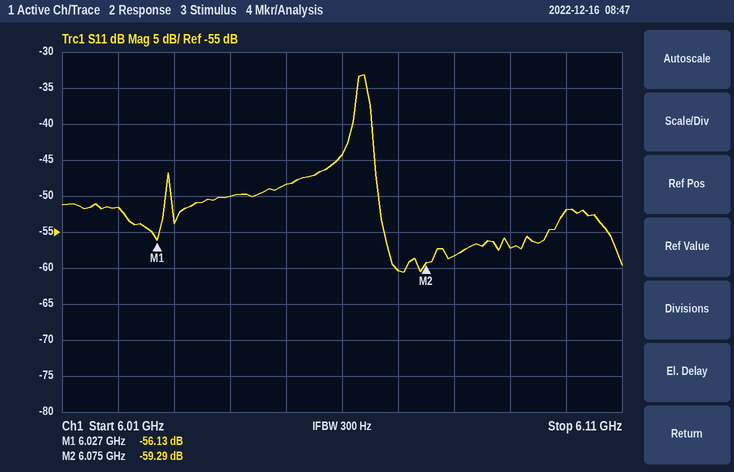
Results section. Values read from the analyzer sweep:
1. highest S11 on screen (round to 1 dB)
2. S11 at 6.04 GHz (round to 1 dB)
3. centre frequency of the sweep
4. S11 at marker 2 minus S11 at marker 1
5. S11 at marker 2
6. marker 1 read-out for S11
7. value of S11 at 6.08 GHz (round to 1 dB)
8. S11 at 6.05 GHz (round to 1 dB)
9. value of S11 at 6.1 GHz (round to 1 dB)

-33 dB
-50 dB
6.06 GHz
-3.16 dB
-59.29 dB
-56.13 dB
-58 dB
-48 dB
-52 dB
